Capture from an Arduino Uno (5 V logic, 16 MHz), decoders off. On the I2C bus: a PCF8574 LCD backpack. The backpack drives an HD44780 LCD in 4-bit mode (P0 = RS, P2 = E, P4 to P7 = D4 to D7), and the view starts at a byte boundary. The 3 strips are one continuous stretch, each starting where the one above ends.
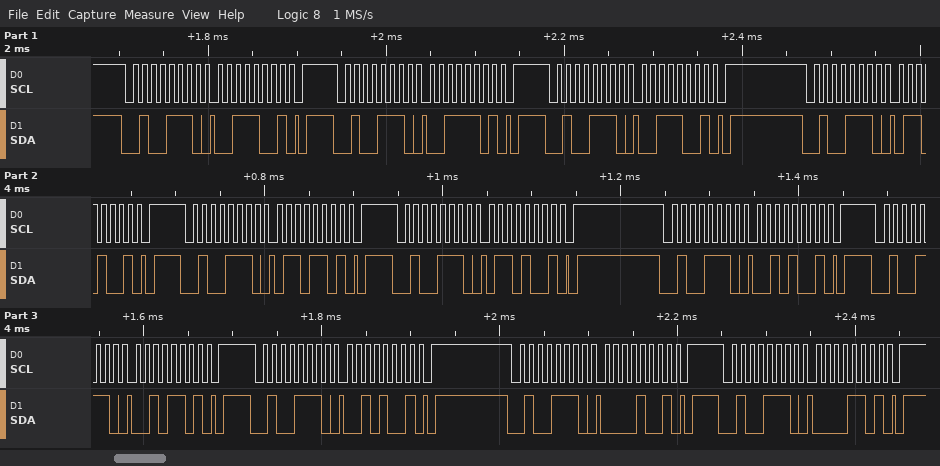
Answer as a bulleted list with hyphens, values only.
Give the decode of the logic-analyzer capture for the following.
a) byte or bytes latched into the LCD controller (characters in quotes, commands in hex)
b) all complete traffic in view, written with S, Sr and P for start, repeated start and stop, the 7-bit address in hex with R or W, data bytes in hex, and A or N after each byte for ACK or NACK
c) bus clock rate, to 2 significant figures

- '6'
- S 27W A 39 A P S 27W A 3D A P S 27W A 39 A P S 27W A 69 A P S 27W A 6D A P S 27W A 69 A P S 27W A 29 A P S 27W A 2D A P S 27W A 29 A P S 27W A 09 A P S 27W A 0D A P
- 100 kHz
